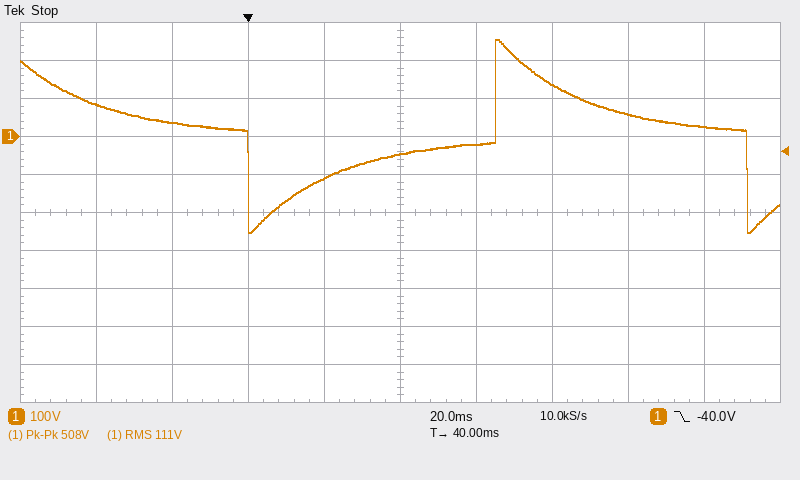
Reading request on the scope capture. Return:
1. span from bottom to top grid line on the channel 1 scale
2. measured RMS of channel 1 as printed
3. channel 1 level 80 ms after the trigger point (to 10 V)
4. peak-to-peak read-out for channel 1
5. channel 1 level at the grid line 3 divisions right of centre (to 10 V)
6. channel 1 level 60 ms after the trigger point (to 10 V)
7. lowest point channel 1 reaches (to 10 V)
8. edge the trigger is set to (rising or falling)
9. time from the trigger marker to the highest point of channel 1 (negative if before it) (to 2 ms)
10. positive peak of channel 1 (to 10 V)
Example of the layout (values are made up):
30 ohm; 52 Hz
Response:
1 kV; 111 V; 140 V; 508 V; 60 V; -20 V; -250 V; falling; +66 ms; 260 V
